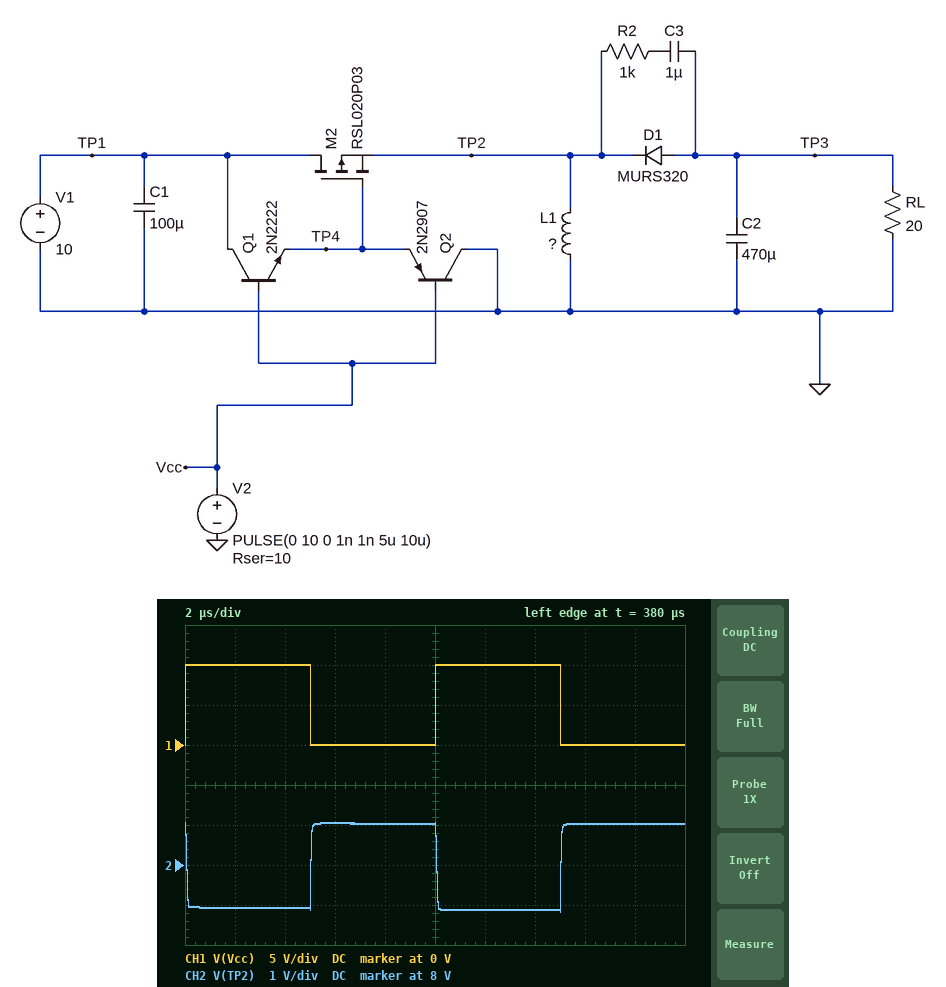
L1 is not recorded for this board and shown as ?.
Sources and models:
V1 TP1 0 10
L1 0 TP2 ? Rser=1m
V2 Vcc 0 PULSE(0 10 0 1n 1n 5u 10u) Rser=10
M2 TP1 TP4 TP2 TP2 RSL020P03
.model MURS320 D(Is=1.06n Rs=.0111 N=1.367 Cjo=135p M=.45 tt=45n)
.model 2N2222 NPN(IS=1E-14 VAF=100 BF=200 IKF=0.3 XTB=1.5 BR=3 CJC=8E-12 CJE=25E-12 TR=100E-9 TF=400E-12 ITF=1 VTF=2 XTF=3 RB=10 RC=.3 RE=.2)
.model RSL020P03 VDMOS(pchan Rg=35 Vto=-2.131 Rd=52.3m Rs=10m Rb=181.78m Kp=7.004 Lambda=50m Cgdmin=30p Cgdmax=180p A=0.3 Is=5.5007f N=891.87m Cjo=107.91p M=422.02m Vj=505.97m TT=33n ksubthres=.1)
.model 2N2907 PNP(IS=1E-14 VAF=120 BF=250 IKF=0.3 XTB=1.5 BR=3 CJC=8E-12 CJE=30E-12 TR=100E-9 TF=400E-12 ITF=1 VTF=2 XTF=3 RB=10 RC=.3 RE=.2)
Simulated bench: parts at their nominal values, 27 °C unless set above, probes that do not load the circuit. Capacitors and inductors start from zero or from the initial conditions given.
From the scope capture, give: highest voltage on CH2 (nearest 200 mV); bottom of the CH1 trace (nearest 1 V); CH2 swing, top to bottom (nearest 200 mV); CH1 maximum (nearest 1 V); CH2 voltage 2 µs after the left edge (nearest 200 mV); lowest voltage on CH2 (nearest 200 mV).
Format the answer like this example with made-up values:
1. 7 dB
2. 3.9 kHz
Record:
1. 9.0 V
2. 0 V
3. 2.2 V
4. 10 V
5. 7.0 V
6. 6.8 V
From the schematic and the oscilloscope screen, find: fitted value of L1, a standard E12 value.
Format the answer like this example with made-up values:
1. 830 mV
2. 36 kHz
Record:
1. 270 µH
